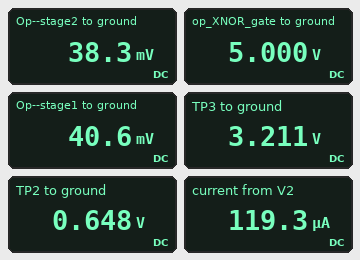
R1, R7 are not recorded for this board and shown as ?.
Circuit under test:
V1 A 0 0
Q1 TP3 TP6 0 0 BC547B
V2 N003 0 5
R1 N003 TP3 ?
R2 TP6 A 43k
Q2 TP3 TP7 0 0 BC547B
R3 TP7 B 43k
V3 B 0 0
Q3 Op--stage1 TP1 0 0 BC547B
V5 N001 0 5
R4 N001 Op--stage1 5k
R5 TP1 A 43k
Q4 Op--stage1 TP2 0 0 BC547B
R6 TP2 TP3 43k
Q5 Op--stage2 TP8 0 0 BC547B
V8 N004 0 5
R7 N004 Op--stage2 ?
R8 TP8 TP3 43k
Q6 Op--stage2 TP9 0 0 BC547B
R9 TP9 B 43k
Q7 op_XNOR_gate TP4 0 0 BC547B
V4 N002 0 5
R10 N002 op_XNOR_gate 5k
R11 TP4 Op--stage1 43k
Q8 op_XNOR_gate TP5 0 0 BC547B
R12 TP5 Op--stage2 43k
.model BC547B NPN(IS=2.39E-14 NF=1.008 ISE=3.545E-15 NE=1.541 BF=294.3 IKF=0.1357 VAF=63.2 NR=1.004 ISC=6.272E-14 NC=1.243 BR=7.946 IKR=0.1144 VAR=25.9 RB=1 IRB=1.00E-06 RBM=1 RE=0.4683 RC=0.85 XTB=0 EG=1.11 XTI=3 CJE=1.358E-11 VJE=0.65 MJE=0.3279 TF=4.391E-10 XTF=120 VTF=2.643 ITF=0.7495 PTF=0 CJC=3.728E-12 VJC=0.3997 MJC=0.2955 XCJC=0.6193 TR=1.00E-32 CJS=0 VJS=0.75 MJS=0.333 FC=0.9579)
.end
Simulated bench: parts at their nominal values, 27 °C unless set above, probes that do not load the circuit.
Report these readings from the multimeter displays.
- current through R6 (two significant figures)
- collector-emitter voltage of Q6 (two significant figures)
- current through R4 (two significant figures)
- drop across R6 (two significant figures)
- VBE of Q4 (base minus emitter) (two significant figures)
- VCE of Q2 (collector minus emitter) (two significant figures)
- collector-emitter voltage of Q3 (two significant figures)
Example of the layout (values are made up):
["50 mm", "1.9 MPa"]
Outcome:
["60 µA", "38 mV", "990 µA", "2.6 V", "650 mV", "3.2 V", "41 mV"]
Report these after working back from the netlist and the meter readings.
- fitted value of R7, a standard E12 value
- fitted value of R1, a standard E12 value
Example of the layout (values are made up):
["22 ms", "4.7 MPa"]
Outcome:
["5.6 kΩ", "15 kΩ"]
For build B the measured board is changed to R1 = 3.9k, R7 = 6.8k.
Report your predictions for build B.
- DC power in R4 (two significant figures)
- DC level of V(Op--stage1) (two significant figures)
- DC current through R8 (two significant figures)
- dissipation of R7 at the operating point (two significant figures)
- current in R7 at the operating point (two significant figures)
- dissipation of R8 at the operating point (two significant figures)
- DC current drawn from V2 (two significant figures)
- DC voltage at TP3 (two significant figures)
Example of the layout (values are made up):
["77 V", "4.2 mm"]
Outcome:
["4.9 mW", "34 mV", "86 µA", "3.6 mW", "730 µA", "320 µW", "170 µA", "4.3 V"]
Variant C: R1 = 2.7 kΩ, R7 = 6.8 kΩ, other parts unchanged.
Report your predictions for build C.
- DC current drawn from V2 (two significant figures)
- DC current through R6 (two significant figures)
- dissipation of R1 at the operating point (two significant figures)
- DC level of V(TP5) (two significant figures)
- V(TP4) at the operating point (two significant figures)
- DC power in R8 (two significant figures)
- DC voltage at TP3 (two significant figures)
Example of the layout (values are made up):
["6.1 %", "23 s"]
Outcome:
["180 µA", "90 µA", "87 µW", "28 mV", "33 mV", "350 µW", "4.5 V"]
